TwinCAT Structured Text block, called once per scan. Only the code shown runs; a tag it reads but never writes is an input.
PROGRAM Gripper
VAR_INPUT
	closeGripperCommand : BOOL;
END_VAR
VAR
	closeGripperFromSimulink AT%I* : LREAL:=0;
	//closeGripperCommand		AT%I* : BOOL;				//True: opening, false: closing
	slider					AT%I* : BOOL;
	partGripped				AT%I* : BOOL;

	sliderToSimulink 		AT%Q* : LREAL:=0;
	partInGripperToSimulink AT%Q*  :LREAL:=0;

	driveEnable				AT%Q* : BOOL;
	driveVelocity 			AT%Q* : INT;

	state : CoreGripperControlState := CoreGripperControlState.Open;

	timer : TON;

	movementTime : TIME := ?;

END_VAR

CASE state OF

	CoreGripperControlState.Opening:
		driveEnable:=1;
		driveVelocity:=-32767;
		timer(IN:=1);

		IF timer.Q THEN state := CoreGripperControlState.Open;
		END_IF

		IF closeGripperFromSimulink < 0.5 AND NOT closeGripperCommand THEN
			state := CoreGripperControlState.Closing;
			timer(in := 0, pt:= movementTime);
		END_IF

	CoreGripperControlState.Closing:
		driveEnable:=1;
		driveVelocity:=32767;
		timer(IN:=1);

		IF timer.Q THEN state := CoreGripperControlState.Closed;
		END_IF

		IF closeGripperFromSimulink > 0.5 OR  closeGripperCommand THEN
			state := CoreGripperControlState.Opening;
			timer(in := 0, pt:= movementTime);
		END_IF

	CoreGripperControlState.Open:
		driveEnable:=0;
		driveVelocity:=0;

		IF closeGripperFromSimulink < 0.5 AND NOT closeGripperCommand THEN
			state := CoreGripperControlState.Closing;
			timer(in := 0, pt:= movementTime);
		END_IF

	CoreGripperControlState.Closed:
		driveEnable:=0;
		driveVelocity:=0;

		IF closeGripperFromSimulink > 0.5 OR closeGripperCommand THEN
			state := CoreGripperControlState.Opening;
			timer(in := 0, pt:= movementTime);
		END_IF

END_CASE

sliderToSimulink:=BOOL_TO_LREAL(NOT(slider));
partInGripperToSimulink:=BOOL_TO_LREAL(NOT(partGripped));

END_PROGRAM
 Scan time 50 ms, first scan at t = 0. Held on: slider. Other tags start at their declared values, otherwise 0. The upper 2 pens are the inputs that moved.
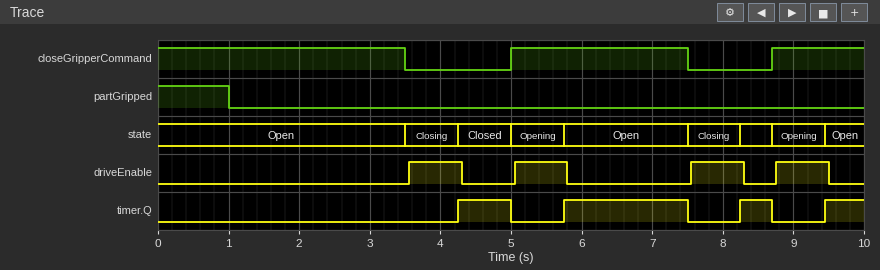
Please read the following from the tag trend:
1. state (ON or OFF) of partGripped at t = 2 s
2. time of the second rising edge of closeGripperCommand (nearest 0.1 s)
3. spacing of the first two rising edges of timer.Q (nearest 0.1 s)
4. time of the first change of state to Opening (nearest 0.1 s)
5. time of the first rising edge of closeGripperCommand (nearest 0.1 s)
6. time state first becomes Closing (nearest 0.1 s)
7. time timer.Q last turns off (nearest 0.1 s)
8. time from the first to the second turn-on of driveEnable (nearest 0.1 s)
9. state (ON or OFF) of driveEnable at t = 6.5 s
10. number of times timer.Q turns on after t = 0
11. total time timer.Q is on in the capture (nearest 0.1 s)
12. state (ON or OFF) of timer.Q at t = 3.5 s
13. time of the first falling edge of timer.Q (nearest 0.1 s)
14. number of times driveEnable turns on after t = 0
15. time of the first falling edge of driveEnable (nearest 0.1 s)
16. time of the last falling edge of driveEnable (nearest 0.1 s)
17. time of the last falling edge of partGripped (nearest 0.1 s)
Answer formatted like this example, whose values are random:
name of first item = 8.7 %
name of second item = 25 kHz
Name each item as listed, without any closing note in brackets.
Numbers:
state (ON or OFF) of partGripped at t = 2 s = OFF
time of the second rising edge of closeGripperCommand = 8.7 s
spacing of the first two rising edges of timer.Q = 1.5 s
time of the first change of state to Opening = 5.0 s
time of the first rising edge of closeGripperCommand = 5.0 s
time state first becomes Closing = 3.5 s
time timer.Q last turns off = 8.7 s
time from the first to the second turn-on of driveEnable = 1.5 s
state (ON or OFF) of driveEnable at t = 6.5 s = OFF
number of times timer.Q turns on after t = 0 = 4
total time timer.Q is on in the capture = 3.5 s
state (ON or OFF) of timer.Q at t = 3.5 s = OFF
time of the first falling edge of timer.Q = 5.0 s
number of times driveEnable turns on after t = 0 = 4
time of the first falling edge of driveEnable = 4.3 s
time of the last falling edge of driveEnable = 9.5 s
time of the last falling edge of partGripped = 1.0 s
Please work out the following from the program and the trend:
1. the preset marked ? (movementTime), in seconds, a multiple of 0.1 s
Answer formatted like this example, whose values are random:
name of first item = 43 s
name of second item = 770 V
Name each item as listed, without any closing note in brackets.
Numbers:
the preset marked ? (movementTime), in seconds, a multiple of 0.1 s = 0.7 s
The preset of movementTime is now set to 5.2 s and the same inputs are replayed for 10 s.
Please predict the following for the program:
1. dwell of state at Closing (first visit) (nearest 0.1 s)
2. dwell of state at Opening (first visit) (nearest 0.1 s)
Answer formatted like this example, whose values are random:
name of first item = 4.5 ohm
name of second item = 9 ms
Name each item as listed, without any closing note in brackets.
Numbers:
dwell of state at Closing (first visit) = 1.5 s
dwell of state at Opening (first visit) = 2.5 s
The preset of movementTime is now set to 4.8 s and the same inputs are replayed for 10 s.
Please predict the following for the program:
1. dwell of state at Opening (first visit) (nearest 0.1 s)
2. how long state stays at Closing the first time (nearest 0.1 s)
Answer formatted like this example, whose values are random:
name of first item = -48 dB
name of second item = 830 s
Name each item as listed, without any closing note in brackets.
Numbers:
dwell of state at Opening (first visit) = 2.5 s
how long state stays at Closing the first time = 1.5 s
